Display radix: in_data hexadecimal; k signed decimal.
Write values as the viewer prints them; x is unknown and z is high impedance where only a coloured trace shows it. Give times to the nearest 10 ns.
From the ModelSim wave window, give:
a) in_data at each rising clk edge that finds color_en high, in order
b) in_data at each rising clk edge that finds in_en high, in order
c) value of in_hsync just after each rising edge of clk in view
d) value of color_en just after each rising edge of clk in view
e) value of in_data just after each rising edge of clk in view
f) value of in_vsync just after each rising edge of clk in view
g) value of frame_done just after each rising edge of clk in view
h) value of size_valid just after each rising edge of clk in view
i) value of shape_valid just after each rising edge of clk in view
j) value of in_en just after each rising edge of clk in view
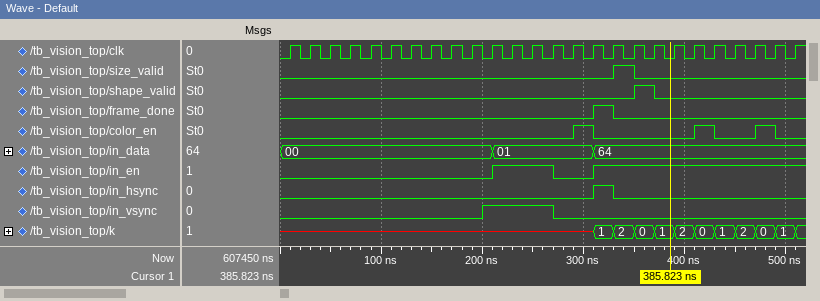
01, 64, 64
01, 01, 01, 64, 64, 64, 64, 64, 64, 64, 64, 64, 64
0 0 0 0 0 0 0 0 0 0 0 0 0 0 0 1 0 0 0 0 0 0 0 0 0 0
0 0 0 0 0 0 0 0 0 0 0 0 0 0 1 0 0 0 0 0 1 0 0 1 0 0
00, 00, 00, 00, 00, 00, 00, 00, 00, 00, 01, 01, 01, 01, 01, 64, 64, 64, 64, 64, 64, 64, 64, 64, 64, 64
0 0 0 0 0 0 0 0 0 0 1 1 1 0 0 0 0 0 0 0 0 0 0 0 0 0
0 0 0 0 0 0 0 0 0 0 0 0 0 0 0 1 0 0 0 0 0 0 0 0 0 0
0 0 0 0 0 0 0 0 0 0 0 0 0 0 0 0 1 0 0 0 0 0 0 0 0 0
0 0 0 0 0 0 0 0 0 0 0 0 0 0 0 0 0 1 0 0 0 0 0 0 0 0
0 0 0 0 0 0 0 0 0 0 1 1 1 0 0 1 1 1 1 1 1 1 1 1 1 1
